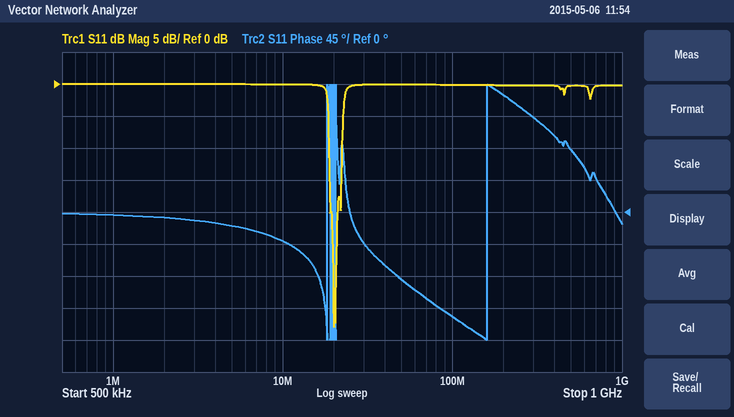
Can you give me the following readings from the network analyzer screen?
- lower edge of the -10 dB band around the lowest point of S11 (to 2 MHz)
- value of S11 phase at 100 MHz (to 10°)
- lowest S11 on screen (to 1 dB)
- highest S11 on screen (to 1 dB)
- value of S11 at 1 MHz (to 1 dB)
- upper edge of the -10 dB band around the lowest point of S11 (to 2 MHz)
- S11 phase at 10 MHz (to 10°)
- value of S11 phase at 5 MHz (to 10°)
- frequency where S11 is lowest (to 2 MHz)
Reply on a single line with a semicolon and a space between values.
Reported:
18 MHz; -150°; -38 dB; 0 dB; 0 dB; 22 MHz; -40°; -20°; 20 MHz
